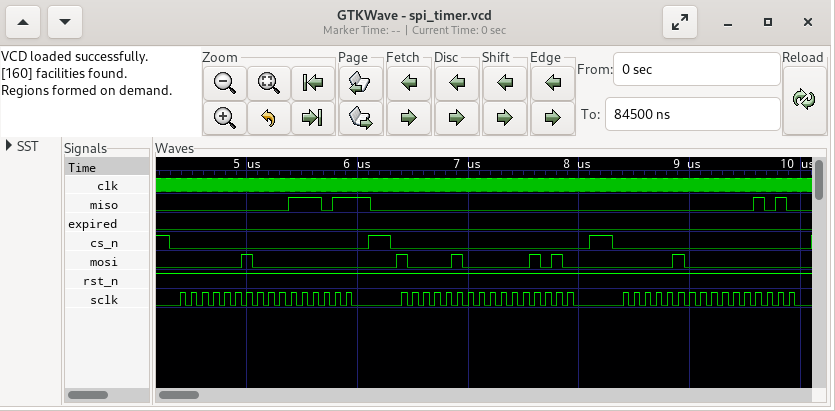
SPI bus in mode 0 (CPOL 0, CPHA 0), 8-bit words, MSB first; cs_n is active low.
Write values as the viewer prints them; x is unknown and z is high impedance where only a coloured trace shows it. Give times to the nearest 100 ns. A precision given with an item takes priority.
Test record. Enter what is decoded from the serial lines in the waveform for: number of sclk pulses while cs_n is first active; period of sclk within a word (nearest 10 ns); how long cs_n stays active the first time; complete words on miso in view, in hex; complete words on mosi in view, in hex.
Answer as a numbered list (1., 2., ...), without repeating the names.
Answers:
1. 16
2. 100 ns
3. 1800 ns
4. 00, 3B, 00, 00, 00, 0A
5. 02, 00, 84, 0A, 04, 00
